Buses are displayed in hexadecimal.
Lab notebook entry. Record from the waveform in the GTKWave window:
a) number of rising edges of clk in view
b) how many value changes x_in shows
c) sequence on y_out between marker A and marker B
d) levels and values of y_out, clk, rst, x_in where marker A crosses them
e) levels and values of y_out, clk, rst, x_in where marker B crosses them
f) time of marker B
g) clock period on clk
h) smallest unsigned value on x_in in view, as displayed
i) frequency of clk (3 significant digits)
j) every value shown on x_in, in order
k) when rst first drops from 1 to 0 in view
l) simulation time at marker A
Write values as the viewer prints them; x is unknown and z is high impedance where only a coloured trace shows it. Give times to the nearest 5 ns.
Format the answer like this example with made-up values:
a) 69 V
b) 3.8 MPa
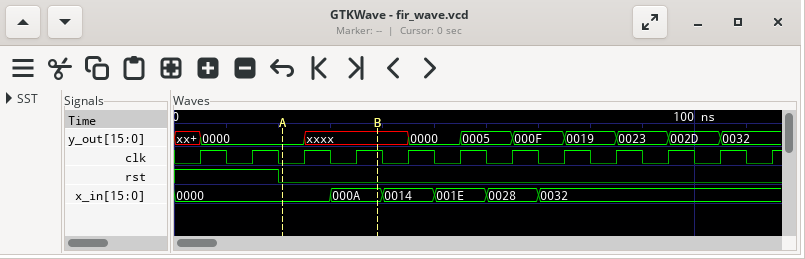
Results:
a) 12
b) 5
c) 0000, xxxx
d) y_out=0000, clk=0, rst=0, x_in=0000
e) y_out=xxxx, clk=1, rst=0, x_in=000A
f) 40 ns
g) 10 ns
h) 0000
i) 100 MHz
j) 0000, 000A, 0014, 001E, 0028, 0032
k) 20 ns
l) 20 ns
